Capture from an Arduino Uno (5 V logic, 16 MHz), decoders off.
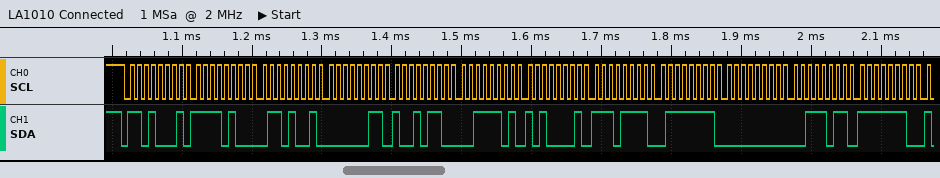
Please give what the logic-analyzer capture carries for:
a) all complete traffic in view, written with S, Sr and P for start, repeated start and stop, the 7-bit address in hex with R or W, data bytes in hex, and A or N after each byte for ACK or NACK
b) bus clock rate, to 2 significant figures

S 68R A F4 A 69 A 03 A 96 A 3D A A1 A EF A 7F A 00 A 3B A FE A
100 kHz
